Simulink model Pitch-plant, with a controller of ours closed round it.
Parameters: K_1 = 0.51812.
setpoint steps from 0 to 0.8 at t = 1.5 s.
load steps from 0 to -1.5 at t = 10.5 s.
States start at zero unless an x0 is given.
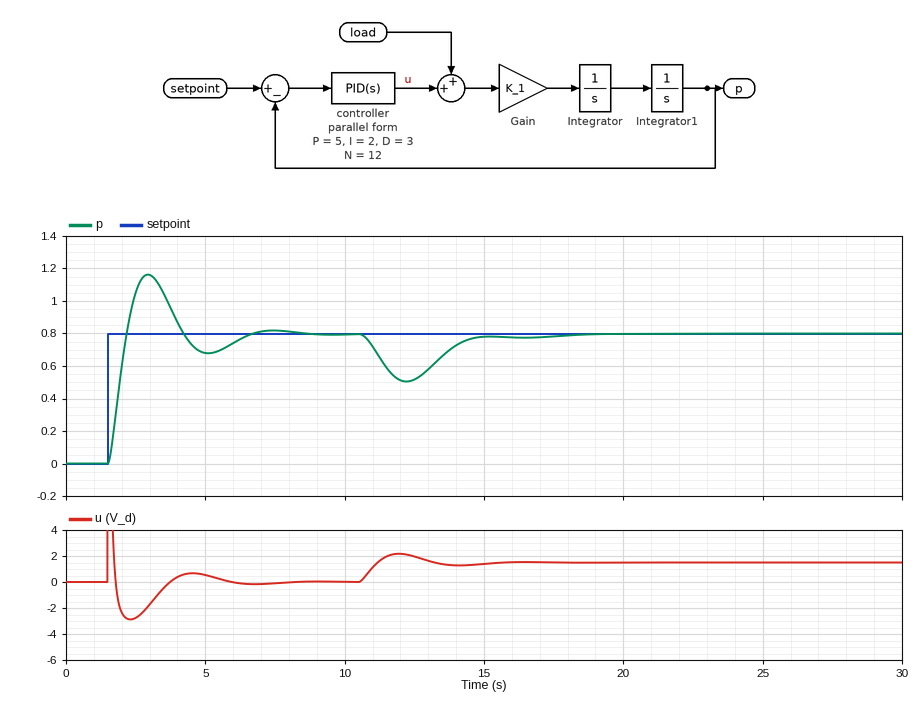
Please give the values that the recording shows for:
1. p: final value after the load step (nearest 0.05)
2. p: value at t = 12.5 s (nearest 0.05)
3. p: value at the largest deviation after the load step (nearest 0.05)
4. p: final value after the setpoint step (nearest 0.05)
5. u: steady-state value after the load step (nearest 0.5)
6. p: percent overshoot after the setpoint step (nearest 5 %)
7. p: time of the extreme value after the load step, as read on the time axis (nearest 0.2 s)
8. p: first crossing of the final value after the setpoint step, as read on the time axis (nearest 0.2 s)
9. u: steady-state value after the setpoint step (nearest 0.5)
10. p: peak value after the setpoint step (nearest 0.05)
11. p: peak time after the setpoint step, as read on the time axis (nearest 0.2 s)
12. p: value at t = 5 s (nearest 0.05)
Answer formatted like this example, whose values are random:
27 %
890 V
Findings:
0.80
0.50
0.50
0.80
1.5
45 %
12.2 s
2.2 s
0.0
1.15
3.0 s
0.70
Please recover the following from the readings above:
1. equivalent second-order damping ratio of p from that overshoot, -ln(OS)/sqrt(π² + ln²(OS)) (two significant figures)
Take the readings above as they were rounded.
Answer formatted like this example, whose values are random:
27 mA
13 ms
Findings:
0.25
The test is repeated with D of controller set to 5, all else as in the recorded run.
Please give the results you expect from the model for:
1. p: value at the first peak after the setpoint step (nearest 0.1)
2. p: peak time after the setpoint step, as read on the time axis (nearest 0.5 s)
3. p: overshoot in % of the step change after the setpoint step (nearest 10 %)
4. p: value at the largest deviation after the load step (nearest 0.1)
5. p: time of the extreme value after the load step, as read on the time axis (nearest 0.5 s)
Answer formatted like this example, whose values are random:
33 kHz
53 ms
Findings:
1.0
2.5 s
30 %
0.6
12.5 s
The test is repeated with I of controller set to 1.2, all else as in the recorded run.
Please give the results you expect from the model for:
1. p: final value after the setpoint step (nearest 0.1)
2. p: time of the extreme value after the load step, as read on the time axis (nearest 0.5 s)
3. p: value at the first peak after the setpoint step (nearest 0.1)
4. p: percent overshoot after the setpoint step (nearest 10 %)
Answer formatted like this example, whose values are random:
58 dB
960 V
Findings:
0.8
12.5 s
1.1
40 %
